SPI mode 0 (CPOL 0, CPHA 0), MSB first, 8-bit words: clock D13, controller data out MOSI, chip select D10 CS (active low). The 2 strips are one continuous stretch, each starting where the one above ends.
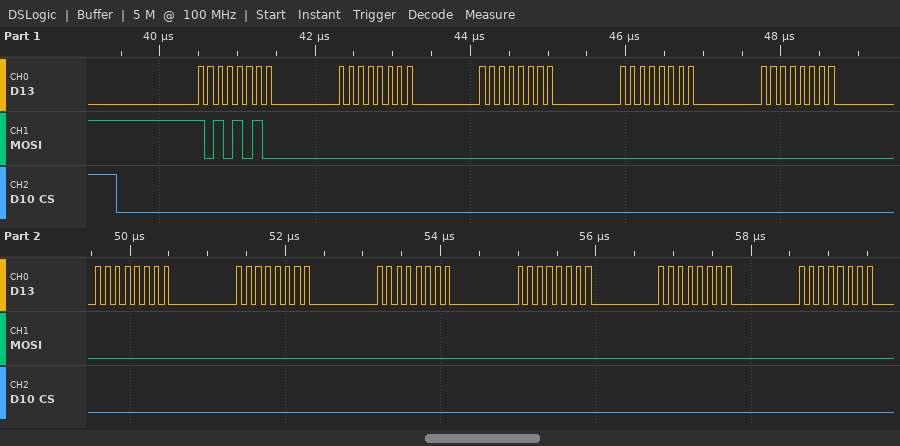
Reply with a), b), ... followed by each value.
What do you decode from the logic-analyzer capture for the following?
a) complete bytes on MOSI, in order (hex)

a) AA 00 00 00 00 00 00 00 00 00 00
